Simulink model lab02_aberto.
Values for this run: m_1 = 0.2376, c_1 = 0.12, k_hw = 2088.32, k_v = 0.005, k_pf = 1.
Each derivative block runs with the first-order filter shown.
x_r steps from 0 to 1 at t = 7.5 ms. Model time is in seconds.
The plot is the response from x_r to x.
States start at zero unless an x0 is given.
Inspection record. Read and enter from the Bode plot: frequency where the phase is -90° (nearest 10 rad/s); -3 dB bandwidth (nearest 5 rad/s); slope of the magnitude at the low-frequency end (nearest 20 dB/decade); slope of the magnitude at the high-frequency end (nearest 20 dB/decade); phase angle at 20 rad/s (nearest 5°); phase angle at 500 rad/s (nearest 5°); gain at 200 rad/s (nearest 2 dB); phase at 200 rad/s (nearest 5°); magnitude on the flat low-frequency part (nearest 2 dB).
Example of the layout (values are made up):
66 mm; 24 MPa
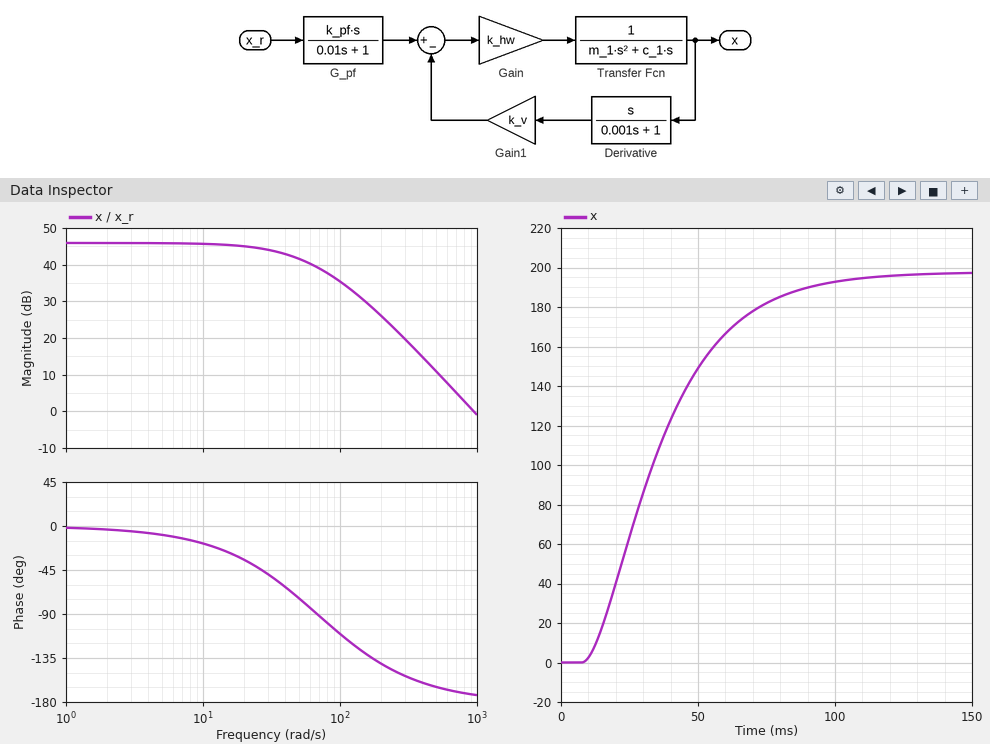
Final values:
70 rad/s; 40 rad/s; 0 dB/decade; -40 dB/decade; -35°; -165°; 26 dB; -140°; 46 dB
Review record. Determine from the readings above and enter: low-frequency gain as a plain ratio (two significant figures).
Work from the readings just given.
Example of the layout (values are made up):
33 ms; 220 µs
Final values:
200
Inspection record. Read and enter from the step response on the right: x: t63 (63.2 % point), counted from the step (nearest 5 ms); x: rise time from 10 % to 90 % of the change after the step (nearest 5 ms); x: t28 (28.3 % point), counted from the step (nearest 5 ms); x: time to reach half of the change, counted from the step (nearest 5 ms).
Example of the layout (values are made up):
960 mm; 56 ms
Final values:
35 ms; 55 ms; 15 ms; 25 ms
